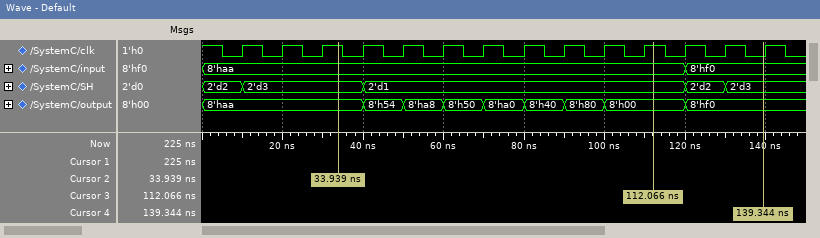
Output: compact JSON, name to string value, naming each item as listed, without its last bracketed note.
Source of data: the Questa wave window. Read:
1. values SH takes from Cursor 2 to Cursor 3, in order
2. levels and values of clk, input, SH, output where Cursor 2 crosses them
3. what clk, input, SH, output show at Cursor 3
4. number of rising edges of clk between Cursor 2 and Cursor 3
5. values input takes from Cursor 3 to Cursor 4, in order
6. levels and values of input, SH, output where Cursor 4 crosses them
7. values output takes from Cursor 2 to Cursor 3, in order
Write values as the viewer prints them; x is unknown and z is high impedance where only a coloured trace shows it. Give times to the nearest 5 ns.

{"values SH takes from Cursor 2 to Cursor 3, in order": "2'd3, 2'd1", "levels and values of clk, input, SH, output where Cursor 2 crosses them": "clk=1, input=8'haa, SH=2'd3, output=8'haa", "what clk, input, SH, output show at Cursor 3": "clk=1, input=8'haa, SH=2'd1, output=8'h00", "number of rising edges of clk between Cursor 2 and Cursor 3": "8", "values input takes from Cursor 3 to Cursor 4, in order": "8'haa, 8'hf0", "levels and values of input, SH, output where Cursor 4 crosses them": "input=8'hf0, SH=2'd3, output=8'hf0", "values output takes from Cursor 2 to Cursor 3, in order": "8'haa, 8'h54, 8'ha8, 8'h50, 8'ha0, 8'h40, 8'h80, 8'h00"}
